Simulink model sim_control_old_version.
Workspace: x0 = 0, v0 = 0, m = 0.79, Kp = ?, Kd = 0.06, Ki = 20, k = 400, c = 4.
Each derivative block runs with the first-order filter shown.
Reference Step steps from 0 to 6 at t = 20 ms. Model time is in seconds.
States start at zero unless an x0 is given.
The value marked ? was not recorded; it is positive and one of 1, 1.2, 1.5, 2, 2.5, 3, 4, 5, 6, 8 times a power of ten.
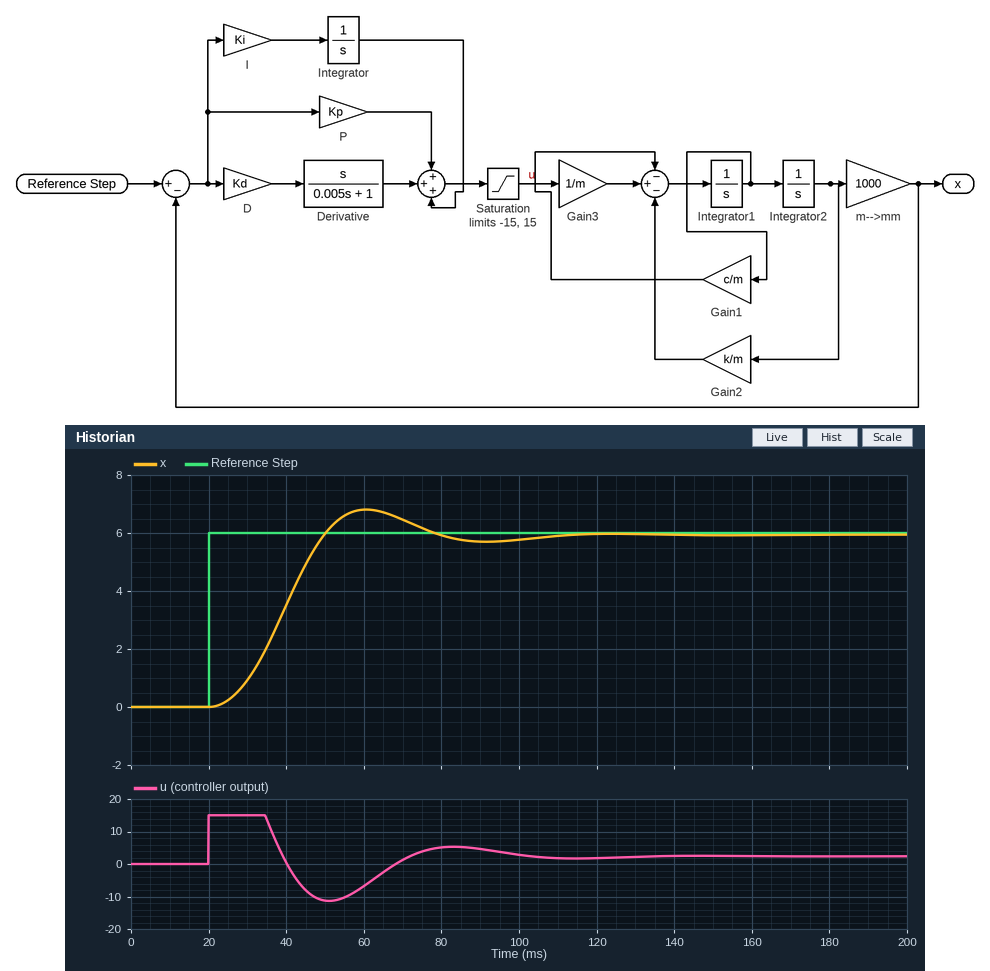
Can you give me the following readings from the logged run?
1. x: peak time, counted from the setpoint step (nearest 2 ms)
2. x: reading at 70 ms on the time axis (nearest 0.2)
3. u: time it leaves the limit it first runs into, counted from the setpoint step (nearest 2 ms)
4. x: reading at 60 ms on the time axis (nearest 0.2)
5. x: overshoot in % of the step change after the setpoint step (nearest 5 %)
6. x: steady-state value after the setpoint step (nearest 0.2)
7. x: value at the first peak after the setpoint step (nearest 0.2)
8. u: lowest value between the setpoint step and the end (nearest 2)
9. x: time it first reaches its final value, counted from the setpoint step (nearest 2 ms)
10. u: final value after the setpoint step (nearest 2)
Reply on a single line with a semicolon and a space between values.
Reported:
40 ms; 6.4; 14 ms; 6.8; 15 %; 6.0; 6.8; -12; 30 ms; 2
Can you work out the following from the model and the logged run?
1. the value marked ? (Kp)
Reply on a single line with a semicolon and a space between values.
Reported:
5
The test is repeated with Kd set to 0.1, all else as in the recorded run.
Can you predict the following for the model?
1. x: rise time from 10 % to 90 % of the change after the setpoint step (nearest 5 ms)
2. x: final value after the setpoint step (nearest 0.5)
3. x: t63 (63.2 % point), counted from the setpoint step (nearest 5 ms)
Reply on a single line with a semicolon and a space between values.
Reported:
25 ms; 6.0; 20 ms
